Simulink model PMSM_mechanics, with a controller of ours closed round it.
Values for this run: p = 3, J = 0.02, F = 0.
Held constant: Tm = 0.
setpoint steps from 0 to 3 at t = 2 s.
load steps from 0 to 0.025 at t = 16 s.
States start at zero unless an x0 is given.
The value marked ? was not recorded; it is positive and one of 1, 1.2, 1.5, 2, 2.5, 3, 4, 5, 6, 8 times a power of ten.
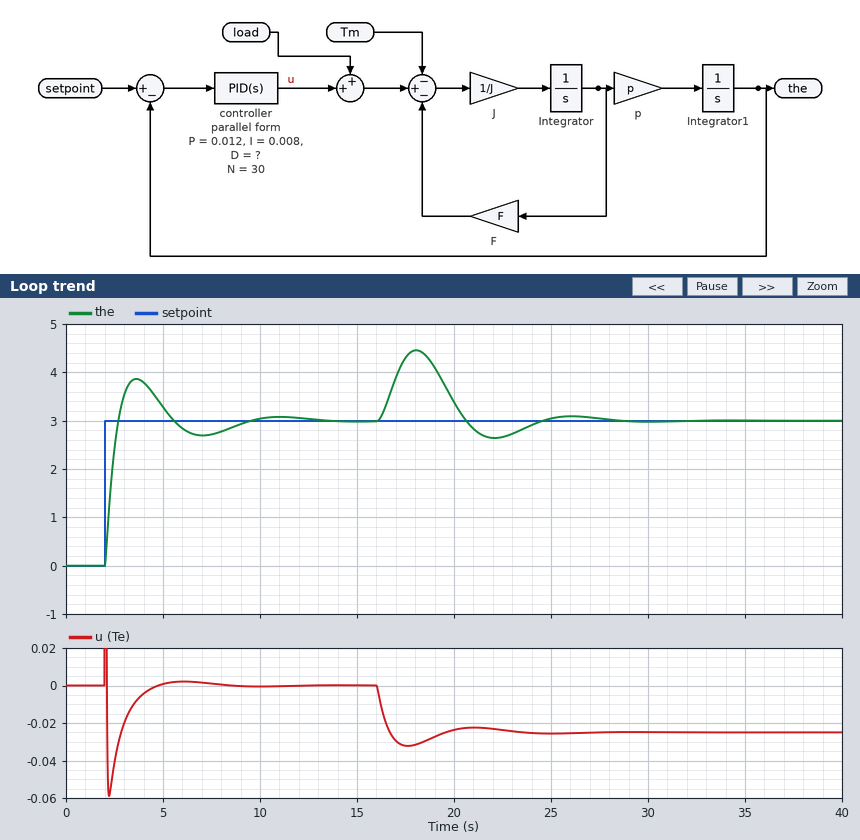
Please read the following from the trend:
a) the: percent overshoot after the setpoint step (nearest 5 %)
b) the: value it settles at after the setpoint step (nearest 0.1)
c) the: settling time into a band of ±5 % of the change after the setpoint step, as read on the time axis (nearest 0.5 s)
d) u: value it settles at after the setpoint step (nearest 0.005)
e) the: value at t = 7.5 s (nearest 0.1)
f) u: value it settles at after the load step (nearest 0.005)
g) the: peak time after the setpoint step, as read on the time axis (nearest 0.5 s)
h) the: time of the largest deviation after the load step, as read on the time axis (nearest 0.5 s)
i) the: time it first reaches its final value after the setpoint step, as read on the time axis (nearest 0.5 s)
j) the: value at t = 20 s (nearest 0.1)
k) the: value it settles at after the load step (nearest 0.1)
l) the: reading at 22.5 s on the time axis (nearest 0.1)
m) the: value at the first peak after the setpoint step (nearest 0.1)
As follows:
30 %
3.0
8.5 s
0.000
2.7
-0.025
3.5 s
18.0 s
2.5 s
3.4
3.0
2.7
3.9
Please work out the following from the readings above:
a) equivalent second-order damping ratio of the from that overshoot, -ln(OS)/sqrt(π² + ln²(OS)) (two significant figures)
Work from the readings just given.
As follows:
0.36
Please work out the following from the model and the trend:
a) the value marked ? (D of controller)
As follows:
0.015
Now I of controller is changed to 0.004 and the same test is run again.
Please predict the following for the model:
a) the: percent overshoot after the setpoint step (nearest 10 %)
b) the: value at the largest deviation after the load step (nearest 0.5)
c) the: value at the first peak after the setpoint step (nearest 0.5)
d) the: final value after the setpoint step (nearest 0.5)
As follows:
20 %
4.5
3.5
3.0
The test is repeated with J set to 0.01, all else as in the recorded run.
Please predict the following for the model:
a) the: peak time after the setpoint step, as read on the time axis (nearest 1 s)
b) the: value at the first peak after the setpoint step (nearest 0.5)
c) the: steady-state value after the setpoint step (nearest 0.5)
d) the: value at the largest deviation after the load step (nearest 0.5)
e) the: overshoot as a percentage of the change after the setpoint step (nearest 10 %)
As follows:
3 s
3.5
3.0
4.5
20 %
